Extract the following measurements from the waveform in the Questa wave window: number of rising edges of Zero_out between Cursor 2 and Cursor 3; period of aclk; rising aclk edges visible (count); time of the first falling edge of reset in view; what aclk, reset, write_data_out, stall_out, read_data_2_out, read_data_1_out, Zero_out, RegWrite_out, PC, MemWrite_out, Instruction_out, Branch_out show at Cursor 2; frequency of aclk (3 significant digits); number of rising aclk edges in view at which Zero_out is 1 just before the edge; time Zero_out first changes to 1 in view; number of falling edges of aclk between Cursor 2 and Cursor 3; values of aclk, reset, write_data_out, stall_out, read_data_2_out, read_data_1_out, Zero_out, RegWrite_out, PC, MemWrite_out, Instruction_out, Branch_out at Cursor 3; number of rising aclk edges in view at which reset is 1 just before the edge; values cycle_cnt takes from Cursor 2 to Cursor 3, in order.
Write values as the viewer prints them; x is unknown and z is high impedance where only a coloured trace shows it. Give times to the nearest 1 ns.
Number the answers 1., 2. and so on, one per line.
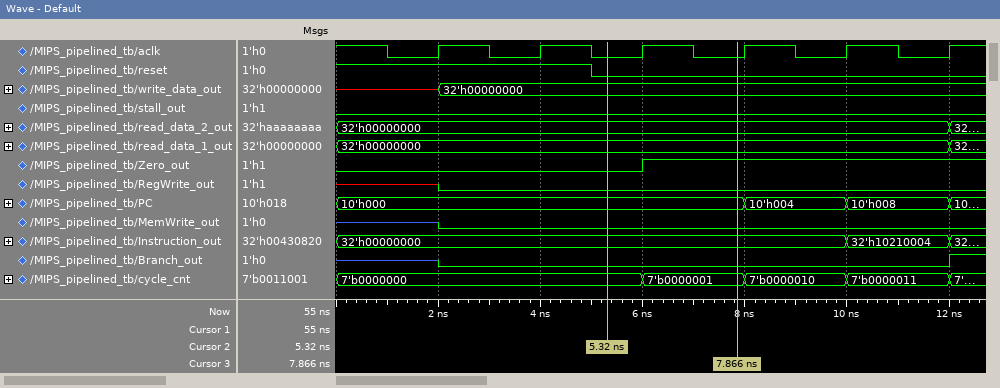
1. 1
2. 2 ns
3. 6
4. 5 ns
5. aclk=0, reset=0, write_data_out=32'h00000000, stall_out=0, read_data_2_out=32'h00000000, read_data_1_out=32'h00000000, Zero_out=0, RegWrite_out=0, PC=10'h000, MemWrite_out=0, Instruction_out=32'h00000000, Branch_out=0
6. 500 MHz
7. 3
8. 6 ns
9. 1
10. aclk=0, reset=0, write_data_out=32'h00000000, stall_out=0, read_data_2_out=32'h00000000, read_data_1_out=32'h00000000, Zero_out=1, RegWrite_out=0, PC=10'h000, MemWrite_out=0, Instruction_out=32'h00000000, Branch_out=0
11. 2
12. 7'b0000000, 7'b0000001
